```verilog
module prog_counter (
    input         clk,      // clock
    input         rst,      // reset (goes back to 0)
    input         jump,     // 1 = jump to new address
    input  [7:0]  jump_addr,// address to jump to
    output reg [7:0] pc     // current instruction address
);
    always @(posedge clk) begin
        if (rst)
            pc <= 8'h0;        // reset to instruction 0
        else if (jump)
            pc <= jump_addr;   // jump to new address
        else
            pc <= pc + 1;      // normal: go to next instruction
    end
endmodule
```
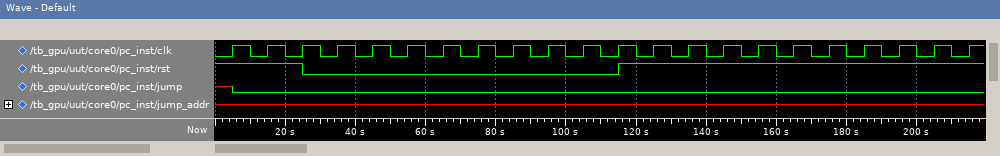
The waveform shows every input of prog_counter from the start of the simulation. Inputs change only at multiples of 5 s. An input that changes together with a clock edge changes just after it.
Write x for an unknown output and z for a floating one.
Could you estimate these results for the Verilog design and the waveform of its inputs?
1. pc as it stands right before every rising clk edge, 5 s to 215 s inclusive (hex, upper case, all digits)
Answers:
x, 00, 00, 00, 01, 02, 03, 04, 05, 06, 07, 08, 09, 00, 00, 00, 00, 00, 00, 00, 00, 00
